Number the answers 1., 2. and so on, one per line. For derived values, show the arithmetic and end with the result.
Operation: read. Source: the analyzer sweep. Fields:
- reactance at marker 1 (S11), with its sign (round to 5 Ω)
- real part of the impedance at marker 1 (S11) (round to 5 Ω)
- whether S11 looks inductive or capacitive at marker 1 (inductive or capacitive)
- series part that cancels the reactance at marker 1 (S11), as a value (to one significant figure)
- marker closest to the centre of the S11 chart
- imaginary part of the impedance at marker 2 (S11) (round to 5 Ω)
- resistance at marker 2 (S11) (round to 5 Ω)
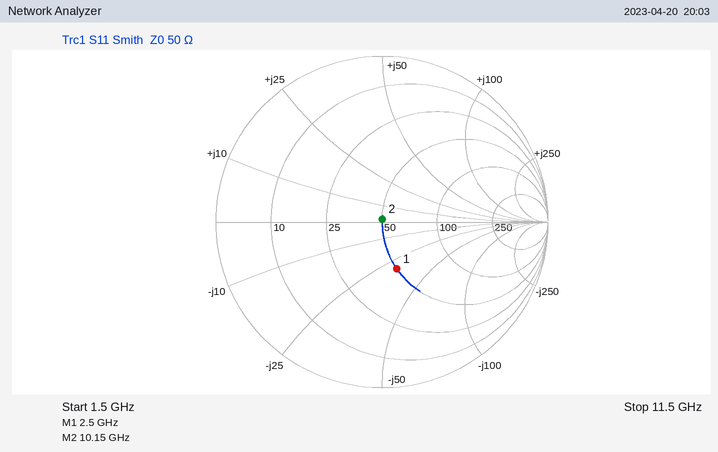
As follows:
1. -30 Ω
2. 50 Ω
3. capacitive
4. L = 30 Ω/(2π × 2.5 GHz) ≈ 2 nH
5. marker 2
6. 0 Ω
7. 50 Ω
